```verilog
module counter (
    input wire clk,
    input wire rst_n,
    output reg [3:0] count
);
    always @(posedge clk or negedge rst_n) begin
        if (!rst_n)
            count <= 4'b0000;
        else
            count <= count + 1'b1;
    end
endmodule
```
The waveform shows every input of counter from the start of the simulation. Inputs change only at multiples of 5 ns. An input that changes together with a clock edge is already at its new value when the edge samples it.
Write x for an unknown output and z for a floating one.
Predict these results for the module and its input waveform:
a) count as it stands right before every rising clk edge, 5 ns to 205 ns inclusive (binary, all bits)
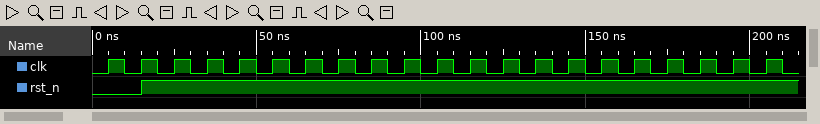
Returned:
0000, 0000, 0001, 0010, 0011, 0100, 0101, 0110, 0111, 1000, 1001, 1010, 1011, 1100, 1101, 1110, 1111, 0000, 0001, 0010, 0011
